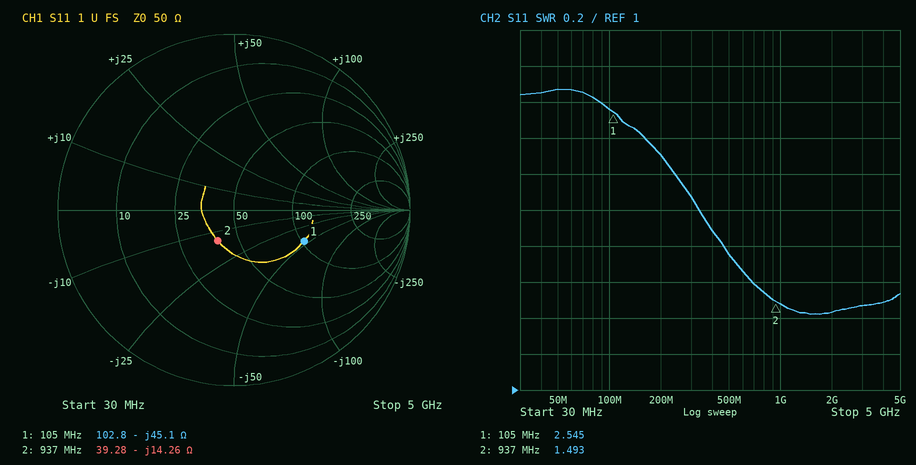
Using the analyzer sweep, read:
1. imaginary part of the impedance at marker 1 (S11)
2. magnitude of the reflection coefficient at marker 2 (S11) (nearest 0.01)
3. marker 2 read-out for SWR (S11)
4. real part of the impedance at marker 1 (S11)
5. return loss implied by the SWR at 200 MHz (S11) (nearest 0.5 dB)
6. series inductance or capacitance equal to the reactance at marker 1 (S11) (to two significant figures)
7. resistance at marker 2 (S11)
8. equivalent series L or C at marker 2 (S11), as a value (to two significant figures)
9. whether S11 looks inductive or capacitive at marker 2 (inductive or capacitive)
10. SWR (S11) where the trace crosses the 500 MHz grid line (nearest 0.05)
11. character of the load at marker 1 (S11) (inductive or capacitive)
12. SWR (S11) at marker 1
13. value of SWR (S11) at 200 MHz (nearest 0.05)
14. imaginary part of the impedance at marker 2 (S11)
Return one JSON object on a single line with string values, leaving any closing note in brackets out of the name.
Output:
{"imaginary part of the impedance at marker 1": "-45.1 Ω", "magnitude of the reflection coefficient at marker 2 (S11)": "0.20", "marker 2 read-out for SWR": "1.493", "real part of the impedance at marker 1": "102.8 Ω", "return loss implied by the SWR at 200 MHz (S11)": "8.0 dB", "series inductance or capacitance equal to the reactance at marker 1 (S11)": "34 pF", "resistance at marker 2": "39.28 Ω", "equivalent series L or C at marker 2 (S11), as a value": "12 pF", "whether S11 looks inductive or capacitive at marker 2": "capacitive", "SWR (S11) where the trace crosses the 500 MHz grid line": "1.75", "character of the load at marker 1 (S11)": "capacitive", "SWR (S11) at marker 1": "2.545", "value of SWR (S11) at 200 MHz": "2.30", "imaginary part of the impedance at marker 2": "-14.26 Ω"}
